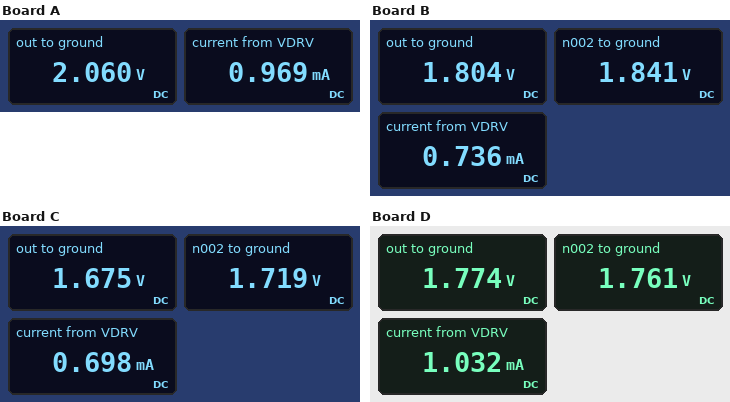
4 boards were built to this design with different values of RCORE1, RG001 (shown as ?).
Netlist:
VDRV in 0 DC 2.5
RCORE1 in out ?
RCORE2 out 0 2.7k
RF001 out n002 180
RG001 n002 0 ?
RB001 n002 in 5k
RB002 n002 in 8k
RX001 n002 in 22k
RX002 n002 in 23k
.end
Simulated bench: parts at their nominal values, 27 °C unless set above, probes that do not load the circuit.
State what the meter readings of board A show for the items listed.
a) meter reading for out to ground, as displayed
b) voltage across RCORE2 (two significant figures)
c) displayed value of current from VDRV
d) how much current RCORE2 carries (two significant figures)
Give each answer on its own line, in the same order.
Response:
2.060 V
2.1 V
0.969 mA
760 µA
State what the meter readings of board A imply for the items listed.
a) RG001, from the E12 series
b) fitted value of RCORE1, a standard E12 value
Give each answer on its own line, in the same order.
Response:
10 kΩ
560 Ω
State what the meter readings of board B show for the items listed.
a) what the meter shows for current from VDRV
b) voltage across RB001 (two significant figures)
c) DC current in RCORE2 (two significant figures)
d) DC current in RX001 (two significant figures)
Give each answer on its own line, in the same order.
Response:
0.736 mA
660 mV
670 µA
30 µA
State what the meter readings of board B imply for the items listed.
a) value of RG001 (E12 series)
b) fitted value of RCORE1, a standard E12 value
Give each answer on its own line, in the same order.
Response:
27 kΩ
1.5 kΩ
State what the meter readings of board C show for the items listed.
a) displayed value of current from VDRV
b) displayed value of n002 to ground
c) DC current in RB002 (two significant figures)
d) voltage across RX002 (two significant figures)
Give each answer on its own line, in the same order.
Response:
0.698 mA
1.719 V
98 µA
780 mV
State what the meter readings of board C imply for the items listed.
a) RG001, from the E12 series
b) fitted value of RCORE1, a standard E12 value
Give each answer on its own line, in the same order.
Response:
22 kΩ
2.2 kΩ
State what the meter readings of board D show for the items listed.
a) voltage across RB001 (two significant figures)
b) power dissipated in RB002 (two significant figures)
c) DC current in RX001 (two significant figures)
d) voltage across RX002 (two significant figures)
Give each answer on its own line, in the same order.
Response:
740 mV
68 µW
34 µA
740 mV
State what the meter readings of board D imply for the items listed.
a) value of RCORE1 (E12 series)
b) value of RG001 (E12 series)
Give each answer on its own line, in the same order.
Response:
1 kΩ
4.7 kΩ
